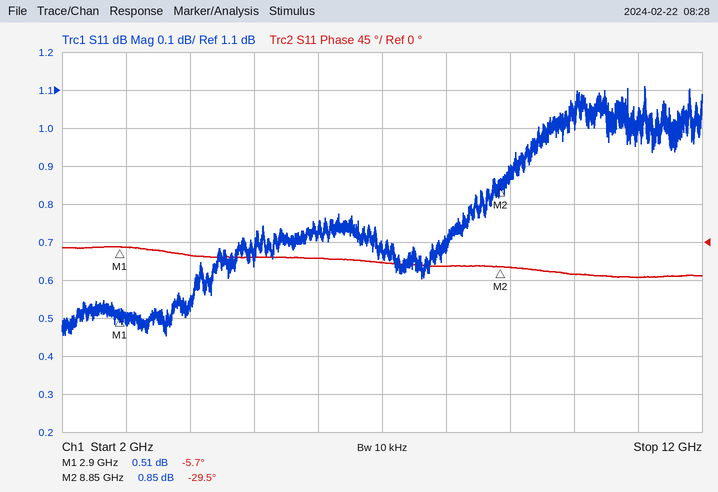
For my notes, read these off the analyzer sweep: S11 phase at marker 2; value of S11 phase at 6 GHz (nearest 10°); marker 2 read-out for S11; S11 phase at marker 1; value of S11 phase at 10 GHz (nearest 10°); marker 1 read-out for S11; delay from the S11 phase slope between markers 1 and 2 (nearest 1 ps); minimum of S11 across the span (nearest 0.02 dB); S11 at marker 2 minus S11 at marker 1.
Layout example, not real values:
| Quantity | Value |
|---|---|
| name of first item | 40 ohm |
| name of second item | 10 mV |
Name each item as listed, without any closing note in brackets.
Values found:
| Quantity | Value |
|---|---|
| S11 phase at marker 2 | -29.5° |
| value of S11 phase at 6 GHz | -20° |
| marker 2 read-out for S11 | 0.85 dB |
| S11 phase at marker 1 | -5.7° |
| value of S11 phase at 10 GHz | -40° |
| marker 1 read-out for S11 | 0.51 dB |
| delay from the S11 phase slope between markers 1 and 2 | 11 ps |
| minimum of S11 across the span | 0.46 dB |
| S11 at marker 2 minus S11 at marker 1 | 0.34 dB |
